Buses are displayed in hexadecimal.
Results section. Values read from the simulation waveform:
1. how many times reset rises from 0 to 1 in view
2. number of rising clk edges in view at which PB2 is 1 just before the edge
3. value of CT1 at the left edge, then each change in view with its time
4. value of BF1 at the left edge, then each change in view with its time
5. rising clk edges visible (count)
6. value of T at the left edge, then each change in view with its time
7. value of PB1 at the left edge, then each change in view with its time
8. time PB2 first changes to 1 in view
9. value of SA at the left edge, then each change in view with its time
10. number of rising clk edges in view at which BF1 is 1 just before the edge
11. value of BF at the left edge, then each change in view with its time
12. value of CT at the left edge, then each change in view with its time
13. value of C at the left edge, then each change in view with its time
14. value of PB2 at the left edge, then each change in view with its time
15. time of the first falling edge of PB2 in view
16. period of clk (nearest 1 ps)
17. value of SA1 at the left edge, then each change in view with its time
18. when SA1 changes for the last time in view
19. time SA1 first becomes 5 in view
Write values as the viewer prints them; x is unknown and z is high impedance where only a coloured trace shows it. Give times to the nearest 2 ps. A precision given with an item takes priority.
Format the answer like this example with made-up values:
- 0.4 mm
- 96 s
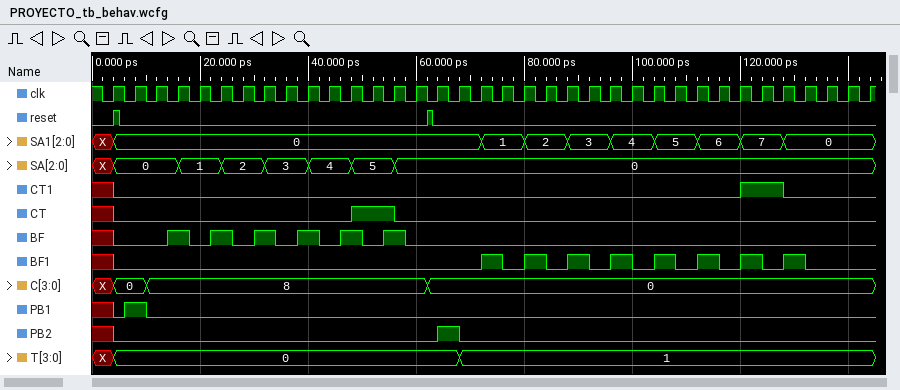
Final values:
- 2
- 1
- x, 0 at 4 ps, 1 at 120 ps, 0 at 128 ps
- x, 0 at 4 ps, 1 at 72 ps, 0 at 76 ps, 1 at 80 ps, 0 at 84 ps, 1 at 88 ps, 0 at 92 ps, 1 at 96 ps, 0 at 100 ps, 1 at 104 ps, 0 at 108 ps, 1 at 112 ps, 0 at 116 ps, 1 at 120 ps, 0 at 124 ps, 1 at 128 ps, 0 at 132 ps
- 36
- X, 0 at 4 ps, 1 at 68 ps
- x, 0 at 4 ps, 1 at 6 ps, 0 at 10 ps
- 64 ps
- X, 0 at 4 ps, 1 at 16 ps, 2 at 24 ps, 3 at 32 ps, 4 at 40 ps, 5 at 48 ps, 0 at 56 ps
- 8
- x, 0 at 4 ps, 1 at 14 ps, 0 at 18 ps, 1 at 22 ps, 0 at 26 ps, 1 at 30 ps, 0 at 34 ps, 1 at 38 ps, 0 at 42 ps, 1 at 46 ps, 0 at 50 ps, 1 at 54 ps, 0 at 58 ps
- x, 0 at 4 ps, 1 at 48 ps, 0 at 56 ps
- X, 0 at 4 ps, 8 at 10 ps, 0 at 62 ps
- x, 0 at 4 ps, 1 at 64 ps, 0 at 68 ps
- 68 ps
- 4 ps
- X, 0 at 4 ps, 1 at 72 ps, 2 at 80 ps, 3 at 88 ps, 4 at 96 ps, 5 at 104 ps, 6 at 112 ps, 7 at 120 ps, 0 at 128 ps
- 128 ps
- 104 ps
